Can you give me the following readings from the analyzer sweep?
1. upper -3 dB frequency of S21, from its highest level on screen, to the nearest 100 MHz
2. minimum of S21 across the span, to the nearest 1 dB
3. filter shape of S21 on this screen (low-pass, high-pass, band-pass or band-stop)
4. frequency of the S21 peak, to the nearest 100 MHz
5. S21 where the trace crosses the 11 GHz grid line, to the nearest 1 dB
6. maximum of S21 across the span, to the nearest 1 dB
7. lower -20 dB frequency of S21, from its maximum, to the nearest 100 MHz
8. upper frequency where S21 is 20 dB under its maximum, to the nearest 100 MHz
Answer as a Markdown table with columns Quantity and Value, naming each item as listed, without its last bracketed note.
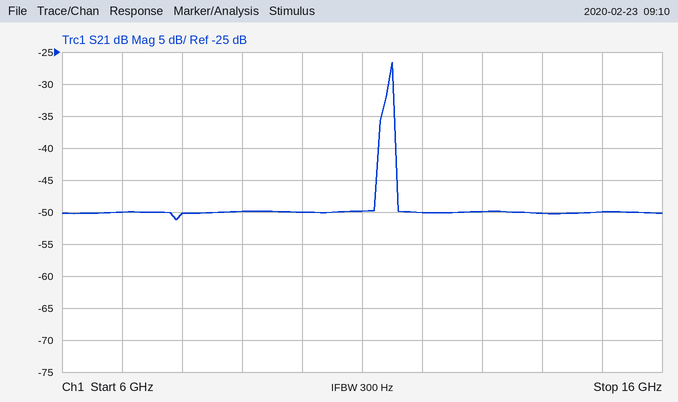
| Quantity | Value |
|---|---|
| upper -3 dB frequency of S21, from its highest level on screen, to the nearest 100 MHz | 11.5 GHz |
| minimum of S21 across the span, to the nearest 1 dB | -51 dB |
| filter shape of S21 on this screen | band-pass |
| frequency of the S21 peak, to the nearest 100 MHz | 11.5 GHz |
| S21 where the trace crosses the 11 GHz grid line, to the nearest 1 dB | -50 dB |
| maximum of S21 across the span, to the nearest 1 dB | -27 dB |
| lower -20 dB frequency of S21, from its maximum, to the nearest 100 MHz | 11.2 GHz |
| upper frequency where S21 is 20 dB under its maximum, to the nearest 100 MHz | 11.6 GHz |
